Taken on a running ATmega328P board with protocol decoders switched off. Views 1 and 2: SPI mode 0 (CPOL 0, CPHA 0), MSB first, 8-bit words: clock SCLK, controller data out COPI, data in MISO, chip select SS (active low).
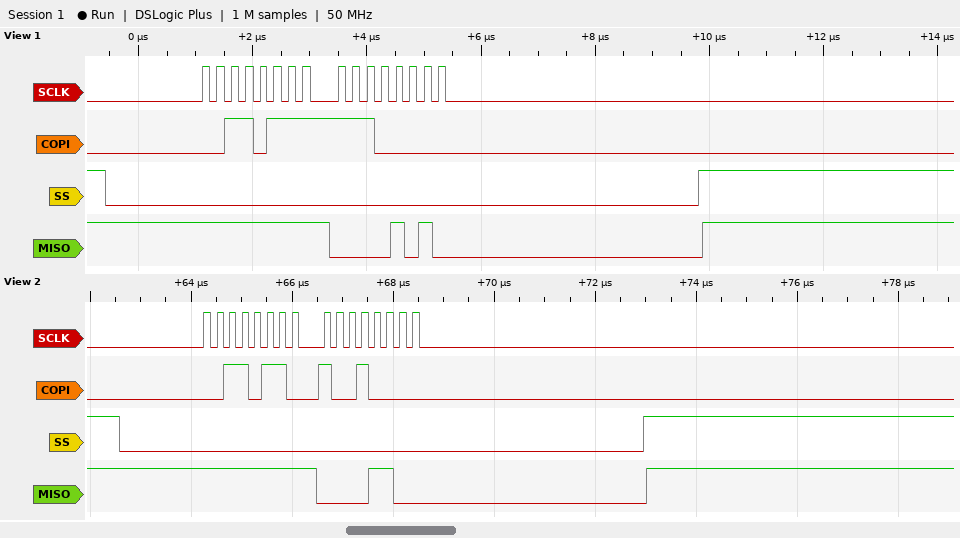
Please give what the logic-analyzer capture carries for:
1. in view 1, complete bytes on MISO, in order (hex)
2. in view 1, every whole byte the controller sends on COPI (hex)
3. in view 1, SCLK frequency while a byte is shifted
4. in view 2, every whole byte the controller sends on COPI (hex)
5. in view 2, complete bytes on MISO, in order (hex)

FF 0A
37 E0
4 MHz
36 90
FF 0C
